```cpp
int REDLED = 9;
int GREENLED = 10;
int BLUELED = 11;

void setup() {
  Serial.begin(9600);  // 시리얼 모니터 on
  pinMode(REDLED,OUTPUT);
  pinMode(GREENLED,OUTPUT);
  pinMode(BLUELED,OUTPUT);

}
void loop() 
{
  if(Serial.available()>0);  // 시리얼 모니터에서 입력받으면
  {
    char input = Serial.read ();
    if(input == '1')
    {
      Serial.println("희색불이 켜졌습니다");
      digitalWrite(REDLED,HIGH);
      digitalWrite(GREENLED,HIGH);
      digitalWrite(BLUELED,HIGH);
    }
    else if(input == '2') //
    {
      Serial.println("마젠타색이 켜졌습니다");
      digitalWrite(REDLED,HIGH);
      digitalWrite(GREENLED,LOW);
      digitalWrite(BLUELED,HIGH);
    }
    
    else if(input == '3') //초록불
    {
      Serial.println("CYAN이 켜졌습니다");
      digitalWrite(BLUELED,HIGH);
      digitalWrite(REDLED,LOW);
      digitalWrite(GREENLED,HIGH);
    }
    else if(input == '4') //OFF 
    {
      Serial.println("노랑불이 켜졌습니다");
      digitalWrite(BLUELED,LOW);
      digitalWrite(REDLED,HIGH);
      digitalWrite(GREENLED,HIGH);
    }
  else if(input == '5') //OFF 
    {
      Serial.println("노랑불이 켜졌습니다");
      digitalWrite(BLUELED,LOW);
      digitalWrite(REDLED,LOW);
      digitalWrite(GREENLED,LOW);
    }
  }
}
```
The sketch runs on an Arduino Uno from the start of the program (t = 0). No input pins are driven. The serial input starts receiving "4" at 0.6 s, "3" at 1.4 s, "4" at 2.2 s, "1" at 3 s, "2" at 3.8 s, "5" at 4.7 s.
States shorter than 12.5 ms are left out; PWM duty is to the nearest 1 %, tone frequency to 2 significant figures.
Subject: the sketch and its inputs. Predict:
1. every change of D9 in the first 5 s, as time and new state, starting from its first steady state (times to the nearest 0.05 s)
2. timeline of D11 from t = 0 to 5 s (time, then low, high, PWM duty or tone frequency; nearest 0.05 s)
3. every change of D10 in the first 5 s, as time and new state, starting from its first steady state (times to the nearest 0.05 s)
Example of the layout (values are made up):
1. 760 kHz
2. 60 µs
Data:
1. 0 s low; 0.6 s high; 1.4 s low; 2.2 s high; 4.7 s low
2. 0 s low; 1.4 s high; 2.2 s low; 3 s high; 4.7 s low
3. 0 s low; 0.6 s high; 3.8 s low
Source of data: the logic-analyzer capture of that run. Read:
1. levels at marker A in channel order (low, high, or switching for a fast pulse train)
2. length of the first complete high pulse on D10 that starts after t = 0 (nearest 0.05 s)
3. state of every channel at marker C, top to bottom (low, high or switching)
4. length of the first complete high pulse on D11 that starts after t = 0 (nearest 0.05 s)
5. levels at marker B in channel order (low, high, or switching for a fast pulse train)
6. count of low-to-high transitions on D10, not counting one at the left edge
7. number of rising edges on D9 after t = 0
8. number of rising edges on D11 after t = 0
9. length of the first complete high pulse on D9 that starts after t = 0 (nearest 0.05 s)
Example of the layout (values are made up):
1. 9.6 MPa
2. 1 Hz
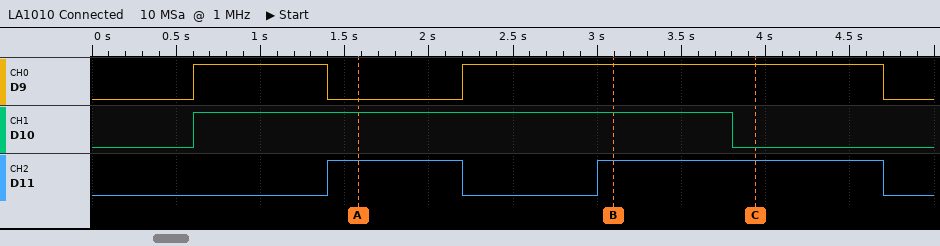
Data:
1. D9 low, D10 high, D11 high
2. 3.20 s
3. D9 high, D10 low, D11 high
4. 0.80 s
5. D9 high, D10 high, D11 high
6. 1
7. 2
8. 2
9. 0.80 s
